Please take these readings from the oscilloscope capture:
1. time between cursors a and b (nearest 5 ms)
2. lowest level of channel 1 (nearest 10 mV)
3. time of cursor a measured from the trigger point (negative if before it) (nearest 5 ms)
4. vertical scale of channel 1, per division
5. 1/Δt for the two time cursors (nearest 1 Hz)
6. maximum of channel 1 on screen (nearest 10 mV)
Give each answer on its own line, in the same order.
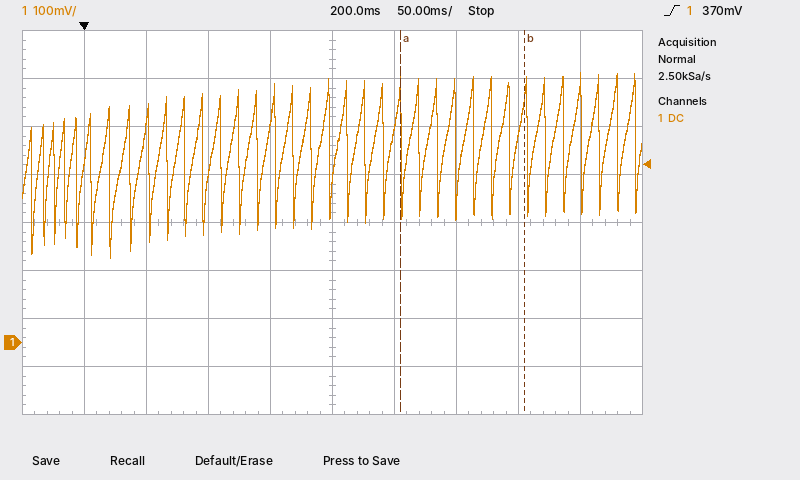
100 ms
180 mV
+255 ms
100 mV
10 Hz
560 mV
